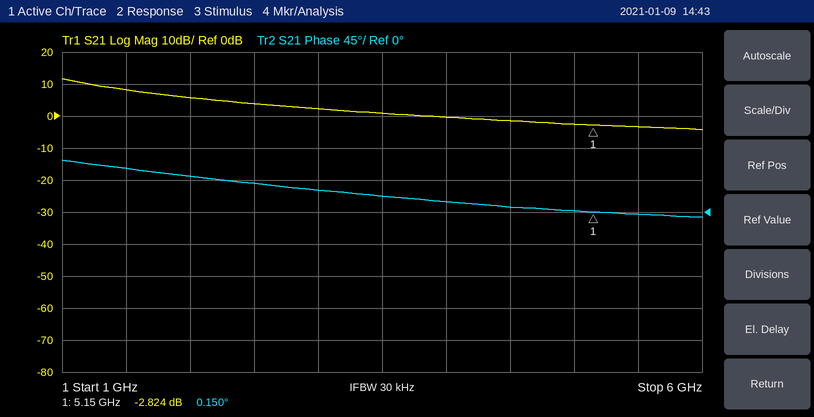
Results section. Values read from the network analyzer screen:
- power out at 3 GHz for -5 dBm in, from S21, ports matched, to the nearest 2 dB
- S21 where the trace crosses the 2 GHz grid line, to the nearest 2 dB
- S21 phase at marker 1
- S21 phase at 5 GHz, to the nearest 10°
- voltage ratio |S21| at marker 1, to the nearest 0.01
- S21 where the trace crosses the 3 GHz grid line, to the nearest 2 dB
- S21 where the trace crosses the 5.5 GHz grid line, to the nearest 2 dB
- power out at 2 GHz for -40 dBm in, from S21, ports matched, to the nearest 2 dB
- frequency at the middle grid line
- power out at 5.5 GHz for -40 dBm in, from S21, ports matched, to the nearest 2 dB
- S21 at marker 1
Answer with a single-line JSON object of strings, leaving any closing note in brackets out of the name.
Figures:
{"power out at 3 GHz for -5 dBm in, from S21, ports matched, to the nearest 2 dB": "-2 dBm", "S21 where the trace crosses the 2 GHz grid line, to the nearest 2 dB": "6 dB", "S21 phase at marker 1": "0.150°", "S21 phase at 5 GHz, to the nearest 10°": "0°", "voltage ratio |S21| at marker 1, to the nearest 0.01": "0.72", "S21 where the trace crosses the 3 GHz grid line, to the nearest 2 dB": "2 dB", "S21 where the trace crosses the 5.5 GHz grid line, to the nearest 2 dB": "-4 dB", "power out at 2 GHz for -40 dBm in, from S21, ports matched, to the nearest 2 dB": "-34 dBm", "frequency at the middle grid line": "3.5 GHz", "power out at 5.5 GHz for -40 dBm in, from S21, ports matched, to the nearest 2 dB": "-44 dBm", "S21 at marker 1": "-2.824 dB"}
